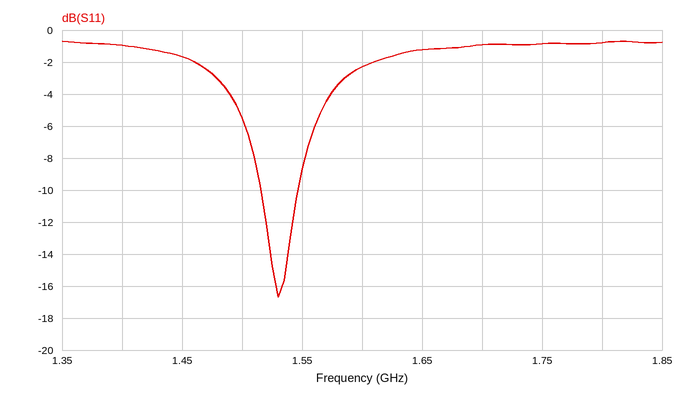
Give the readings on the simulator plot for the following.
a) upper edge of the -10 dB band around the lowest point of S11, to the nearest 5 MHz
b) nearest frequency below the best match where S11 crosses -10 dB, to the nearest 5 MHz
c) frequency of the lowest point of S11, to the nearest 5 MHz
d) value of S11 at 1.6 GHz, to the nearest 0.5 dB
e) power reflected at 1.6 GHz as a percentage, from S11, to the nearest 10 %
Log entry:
1.545 GHz
1.515 GHz
1.530 GHz
-2.5 dB
60 %
